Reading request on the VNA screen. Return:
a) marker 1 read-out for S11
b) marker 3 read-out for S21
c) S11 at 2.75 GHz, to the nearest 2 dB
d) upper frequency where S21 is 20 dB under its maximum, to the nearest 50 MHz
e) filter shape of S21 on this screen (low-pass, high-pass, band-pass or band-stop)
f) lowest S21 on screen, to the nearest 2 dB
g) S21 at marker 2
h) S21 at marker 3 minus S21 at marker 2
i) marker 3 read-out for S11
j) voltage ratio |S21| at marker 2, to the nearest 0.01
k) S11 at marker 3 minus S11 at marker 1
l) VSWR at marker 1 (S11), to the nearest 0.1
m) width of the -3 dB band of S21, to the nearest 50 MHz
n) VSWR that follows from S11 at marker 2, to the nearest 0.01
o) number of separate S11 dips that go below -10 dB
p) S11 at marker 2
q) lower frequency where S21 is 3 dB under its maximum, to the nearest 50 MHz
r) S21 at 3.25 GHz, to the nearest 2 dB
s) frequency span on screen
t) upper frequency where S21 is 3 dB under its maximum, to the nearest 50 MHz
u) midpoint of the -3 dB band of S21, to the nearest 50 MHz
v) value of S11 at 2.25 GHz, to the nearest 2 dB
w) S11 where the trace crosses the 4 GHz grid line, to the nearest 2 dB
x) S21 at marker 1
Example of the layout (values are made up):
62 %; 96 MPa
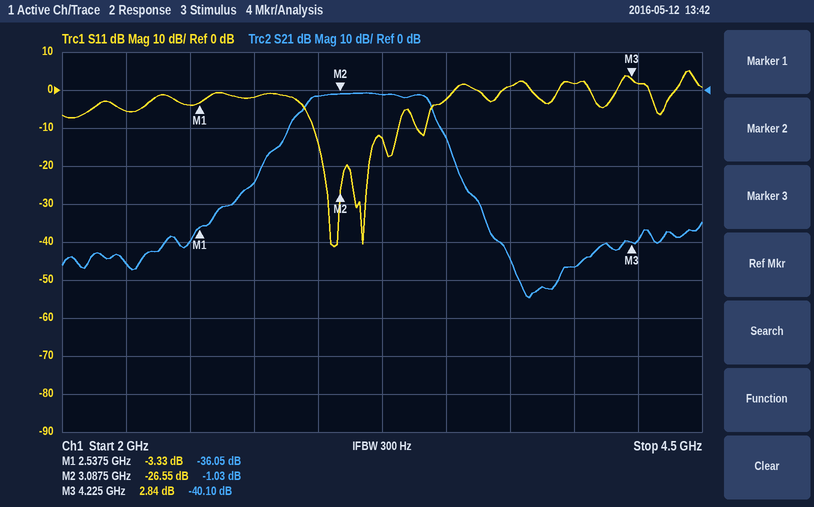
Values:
-3.33 dB; -40.10 dB; -2 dB; 3.55 GHz; band-pass; -54 dB; -1.03 dB; -39.07 dB; 2.84 dB; 0.89; 6.17 dB; 5.3; 500 MHz; 1.10; 4; -26.55 dB; 2.95 GHz; -2 dB; 2.5 GHz; 3.45 GHz; 3.20 GHz; -6 dB; 2 dB; -36.05 dB
